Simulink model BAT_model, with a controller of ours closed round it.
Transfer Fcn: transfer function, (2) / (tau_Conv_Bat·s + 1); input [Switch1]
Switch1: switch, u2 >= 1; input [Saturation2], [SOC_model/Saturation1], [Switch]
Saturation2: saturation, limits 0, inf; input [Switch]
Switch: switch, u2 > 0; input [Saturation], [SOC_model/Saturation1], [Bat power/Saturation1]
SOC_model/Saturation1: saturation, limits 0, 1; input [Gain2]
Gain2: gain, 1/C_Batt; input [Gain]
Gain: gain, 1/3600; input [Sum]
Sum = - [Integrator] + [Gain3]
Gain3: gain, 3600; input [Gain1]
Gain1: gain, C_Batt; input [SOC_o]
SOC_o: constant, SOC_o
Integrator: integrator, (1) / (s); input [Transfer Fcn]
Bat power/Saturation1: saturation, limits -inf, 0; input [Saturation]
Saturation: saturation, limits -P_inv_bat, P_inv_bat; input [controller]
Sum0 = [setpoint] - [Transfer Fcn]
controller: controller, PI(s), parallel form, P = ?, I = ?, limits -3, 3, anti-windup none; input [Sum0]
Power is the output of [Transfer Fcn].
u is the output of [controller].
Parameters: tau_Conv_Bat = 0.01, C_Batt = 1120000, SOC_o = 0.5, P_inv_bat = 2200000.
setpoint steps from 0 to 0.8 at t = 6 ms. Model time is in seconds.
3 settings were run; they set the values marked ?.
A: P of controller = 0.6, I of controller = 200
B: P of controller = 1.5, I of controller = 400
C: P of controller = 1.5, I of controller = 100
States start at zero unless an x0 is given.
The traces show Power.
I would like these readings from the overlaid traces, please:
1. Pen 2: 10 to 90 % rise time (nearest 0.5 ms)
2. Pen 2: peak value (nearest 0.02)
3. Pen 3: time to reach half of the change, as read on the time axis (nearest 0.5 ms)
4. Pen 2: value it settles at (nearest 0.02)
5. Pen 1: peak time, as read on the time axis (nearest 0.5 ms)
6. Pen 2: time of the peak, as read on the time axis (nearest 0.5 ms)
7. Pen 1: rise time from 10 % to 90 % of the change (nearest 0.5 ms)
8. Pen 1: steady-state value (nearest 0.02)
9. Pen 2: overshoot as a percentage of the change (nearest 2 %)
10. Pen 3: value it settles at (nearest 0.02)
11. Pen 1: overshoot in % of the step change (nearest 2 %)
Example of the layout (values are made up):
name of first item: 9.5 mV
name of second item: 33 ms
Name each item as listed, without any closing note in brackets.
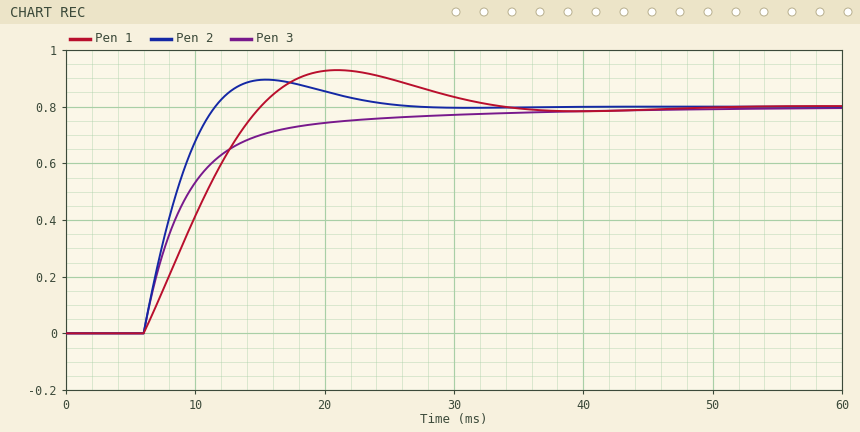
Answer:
Pen 2: 10 to 90 % rise time: 4.0 ms
Pen 2: peak value: 0.90
Pen 3: time to reach half of the change, as read on the time axis: 8.5 ms
Pen 2: value it settles at: 0.80
Pen 1: peak time, as read on the time axis: 21.0 ms
Pen 2: time of the peak, as read on the time axis: 15.5 ms
Pen 1: rise time from 10 % to 90 % of the change: 7.0 ms
Pen 1: steady-state value: 0.80
Pen 2: overshoot as a percentage of the change: 12 %
Pen 3: value it settles at: 0.80
Pen 1: overshoot in % of the step change: 16 %
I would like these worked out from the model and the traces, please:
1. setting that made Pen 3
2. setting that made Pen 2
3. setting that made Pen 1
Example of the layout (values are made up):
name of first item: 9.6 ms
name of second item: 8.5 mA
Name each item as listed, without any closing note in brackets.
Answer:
setting that made Pen 3: C
setting that made Pen 2: B
setting that made Pen 1: A
